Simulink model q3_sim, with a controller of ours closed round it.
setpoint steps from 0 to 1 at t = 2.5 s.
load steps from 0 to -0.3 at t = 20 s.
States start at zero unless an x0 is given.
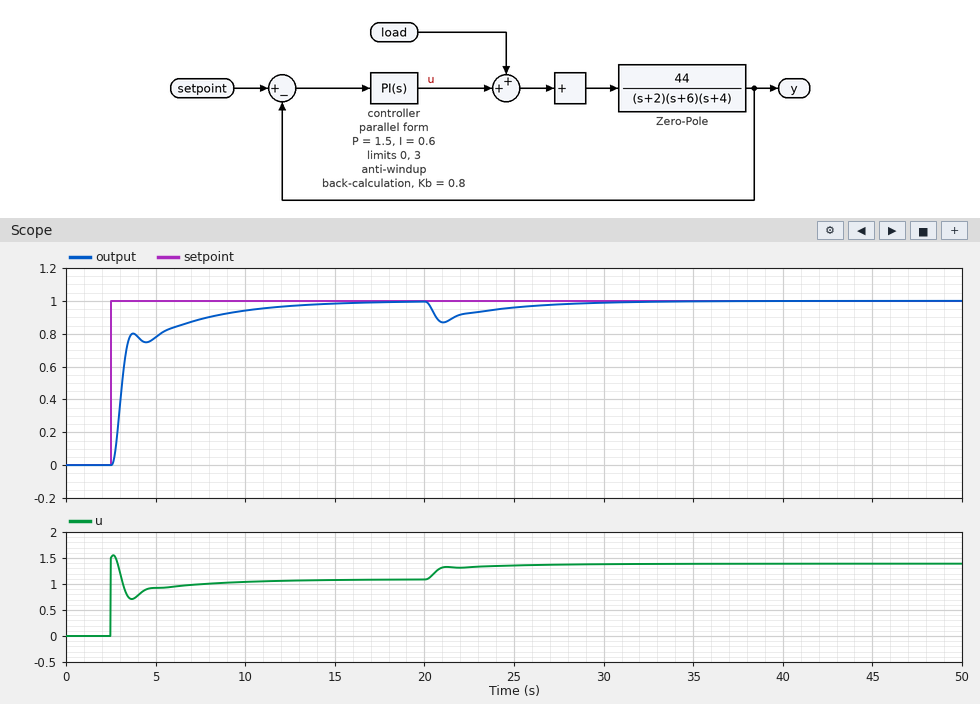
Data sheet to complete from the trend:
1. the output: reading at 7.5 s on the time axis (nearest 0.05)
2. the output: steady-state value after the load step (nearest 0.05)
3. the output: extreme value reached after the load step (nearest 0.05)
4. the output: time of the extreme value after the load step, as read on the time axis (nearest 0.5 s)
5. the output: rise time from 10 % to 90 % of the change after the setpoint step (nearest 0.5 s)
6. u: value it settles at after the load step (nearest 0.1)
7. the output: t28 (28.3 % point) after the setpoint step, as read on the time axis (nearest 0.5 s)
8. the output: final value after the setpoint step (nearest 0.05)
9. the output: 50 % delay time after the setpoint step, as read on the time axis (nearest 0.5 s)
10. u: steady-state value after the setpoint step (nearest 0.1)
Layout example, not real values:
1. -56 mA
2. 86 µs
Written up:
1. 0.90
2. 1.00
3. 0.85
4. 21.0 s
5. 5.0 s
6. 1.4
7. 3.0 s
8. 1.00
9. 3.0 s
10. 1.1
